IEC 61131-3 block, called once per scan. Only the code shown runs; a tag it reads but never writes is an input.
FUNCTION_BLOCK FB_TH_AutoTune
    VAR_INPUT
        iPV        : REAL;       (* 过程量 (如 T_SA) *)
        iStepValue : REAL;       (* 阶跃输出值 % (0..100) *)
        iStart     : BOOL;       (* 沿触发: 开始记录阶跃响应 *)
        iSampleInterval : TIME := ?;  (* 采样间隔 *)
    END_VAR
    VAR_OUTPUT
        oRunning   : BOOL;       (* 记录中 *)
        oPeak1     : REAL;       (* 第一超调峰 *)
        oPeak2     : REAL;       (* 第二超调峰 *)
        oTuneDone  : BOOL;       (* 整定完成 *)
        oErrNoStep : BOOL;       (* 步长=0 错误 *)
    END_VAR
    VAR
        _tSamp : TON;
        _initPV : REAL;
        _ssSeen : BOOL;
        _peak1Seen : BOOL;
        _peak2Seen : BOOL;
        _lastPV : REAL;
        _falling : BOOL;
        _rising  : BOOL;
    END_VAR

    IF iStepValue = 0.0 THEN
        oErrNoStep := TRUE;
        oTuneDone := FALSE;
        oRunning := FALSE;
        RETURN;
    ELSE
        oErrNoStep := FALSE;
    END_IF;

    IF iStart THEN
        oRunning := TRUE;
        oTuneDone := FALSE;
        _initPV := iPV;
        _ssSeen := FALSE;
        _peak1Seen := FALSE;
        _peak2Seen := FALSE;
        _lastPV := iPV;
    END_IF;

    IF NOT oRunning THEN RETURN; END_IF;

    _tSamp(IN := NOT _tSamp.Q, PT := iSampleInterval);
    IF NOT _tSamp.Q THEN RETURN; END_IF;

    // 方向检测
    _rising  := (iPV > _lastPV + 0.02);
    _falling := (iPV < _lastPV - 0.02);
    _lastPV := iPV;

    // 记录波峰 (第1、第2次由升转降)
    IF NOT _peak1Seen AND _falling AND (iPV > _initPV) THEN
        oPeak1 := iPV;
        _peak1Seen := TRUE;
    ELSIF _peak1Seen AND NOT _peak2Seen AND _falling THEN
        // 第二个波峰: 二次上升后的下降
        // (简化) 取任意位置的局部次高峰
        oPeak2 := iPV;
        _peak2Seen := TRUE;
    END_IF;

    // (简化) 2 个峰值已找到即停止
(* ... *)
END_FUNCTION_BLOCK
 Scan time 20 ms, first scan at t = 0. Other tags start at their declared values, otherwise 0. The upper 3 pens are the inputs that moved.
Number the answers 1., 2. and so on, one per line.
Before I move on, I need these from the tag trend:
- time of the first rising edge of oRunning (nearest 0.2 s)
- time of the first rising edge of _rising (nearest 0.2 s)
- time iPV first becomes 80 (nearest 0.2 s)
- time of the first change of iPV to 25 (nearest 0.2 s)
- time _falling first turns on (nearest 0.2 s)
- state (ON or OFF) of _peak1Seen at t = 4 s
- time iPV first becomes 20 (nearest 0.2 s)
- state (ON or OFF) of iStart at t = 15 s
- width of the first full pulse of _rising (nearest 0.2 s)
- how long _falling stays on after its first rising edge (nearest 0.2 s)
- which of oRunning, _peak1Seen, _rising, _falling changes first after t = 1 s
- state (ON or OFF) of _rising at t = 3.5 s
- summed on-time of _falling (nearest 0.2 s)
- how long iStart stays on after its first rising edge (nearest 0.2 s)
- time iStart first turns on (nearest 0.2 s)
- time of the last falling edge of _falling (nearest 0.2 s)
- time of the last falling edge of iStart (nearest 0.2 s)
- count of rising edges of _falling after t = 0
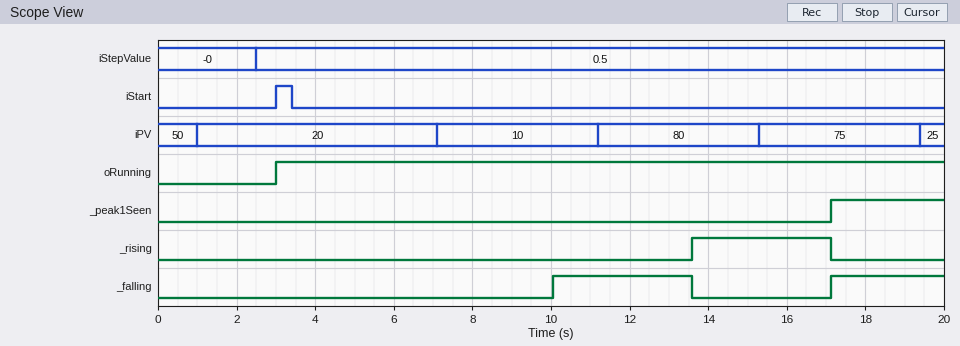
1. 3.0 s
2. 13.6 s
3. 11.2 s
4. 19.4 s
5. 10.0 s
6. OFF
7. 1.0 s
8. OFF
9. 3.6 s
10. 3.6 s
11. oRunning
12. OFF
13. 6.4 s
14. 0.4 s
15. 3.0 s
16. 13.6 s
17. 3.4 s
18. 2
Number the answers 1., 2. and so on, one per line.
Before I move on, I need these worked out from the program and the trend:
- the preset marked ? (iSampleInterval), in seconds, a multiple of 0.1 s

1. 3.5 s
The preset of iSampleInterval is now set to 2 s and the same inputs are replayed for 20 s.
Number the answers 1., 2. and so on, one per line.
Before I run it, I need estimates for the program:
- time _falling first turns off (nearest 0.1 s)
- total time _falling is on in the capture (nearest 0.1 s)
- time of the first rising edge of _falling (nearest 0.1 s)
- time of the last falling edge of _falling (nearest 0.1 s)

1. 11.1 s
2. 4.1 s
3. 9.1 s
4. 19.3 s
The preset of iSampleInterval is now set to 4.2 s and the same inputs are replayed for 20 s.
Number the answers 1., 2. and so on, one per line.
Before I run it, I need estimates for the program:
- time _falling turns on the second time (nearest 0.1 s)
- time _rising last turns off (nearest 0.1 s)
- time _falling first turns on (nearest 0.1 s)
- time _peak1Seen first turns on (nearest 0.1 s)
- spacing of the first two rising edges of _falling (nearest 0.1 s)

1. 15.7 s
2. 15.7 s
3. 7.2 s
4. 15.7 s
5. 8.5 s
